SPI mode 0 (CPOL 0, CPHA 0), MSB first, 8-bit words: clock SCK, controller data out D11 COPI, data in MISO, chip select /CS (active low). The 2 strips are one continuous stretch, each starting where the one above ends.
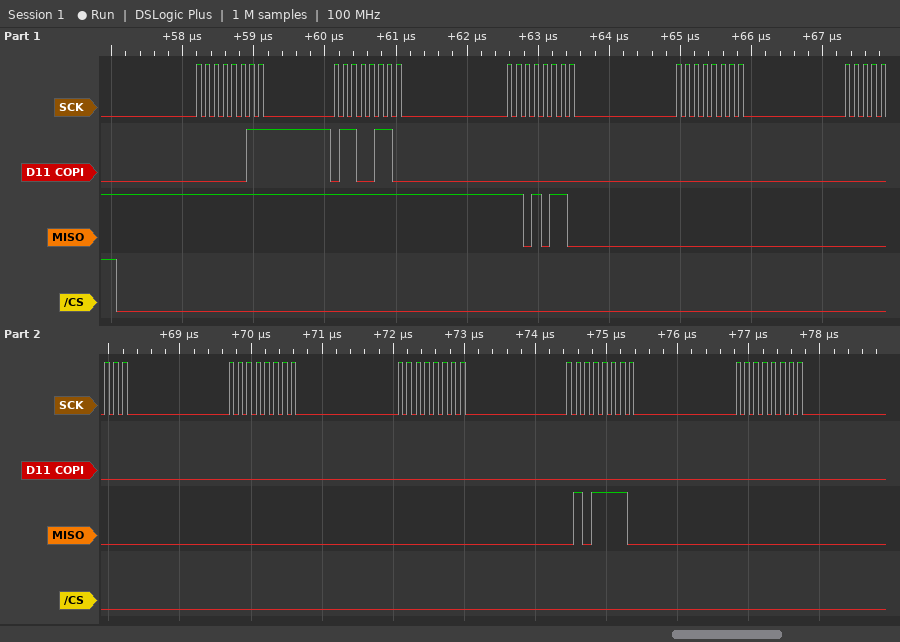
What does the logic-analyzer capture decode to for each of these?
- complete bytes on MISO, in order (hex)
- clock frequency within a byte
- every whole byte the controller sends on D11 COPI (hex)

FF FF D6 00 00 00 00 5E 00
8 MHz
03 66 00 00 00 00 00 00 00
